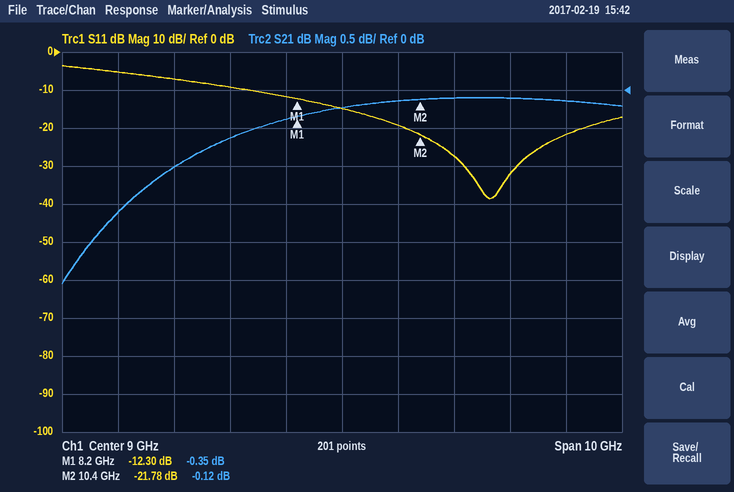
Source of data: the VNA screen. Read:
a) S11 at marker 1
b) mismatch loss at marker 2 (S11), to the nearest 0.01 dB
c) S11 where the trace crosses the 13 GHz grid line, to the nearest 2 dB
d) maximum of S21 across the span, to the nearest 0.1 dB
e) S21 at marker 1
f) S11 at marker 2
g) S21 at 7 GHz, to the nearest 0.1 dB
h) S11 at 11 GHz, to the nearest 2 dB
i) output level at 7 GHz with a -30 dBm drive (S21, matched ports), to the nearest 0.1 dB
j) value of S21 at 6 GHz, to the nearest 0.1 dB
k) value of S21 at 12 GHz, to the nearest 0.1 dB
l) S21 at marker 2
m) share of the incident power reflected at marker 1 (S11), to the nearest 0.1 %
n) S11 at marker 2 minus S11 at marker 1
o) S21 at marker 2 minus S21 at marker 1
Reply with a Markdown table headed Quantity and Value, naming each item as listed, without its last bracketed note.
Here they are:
| Quantity | Value |
|---|---|
| S11 at marker 1 | -12.30 dB |
| mismatch loss at marker 2 (S11), to the nearest 0.01 dB | 0.03 dB |
| S11 where the trace crosses the 13 GHz grid line, to the nearest 2 dB | -22 dB |
| maximum of S21 across the span, to the nearest 0.1 dB | -0.1 dB |
| S21 at marker 1 | -0.35 dB |
| S11 at marker 2 | -21.78 dB |
| S21 at 7 GHz, to the nearest 0.1 dB | -0.6 dB |
| S11 at 11 GHz, to the nearest 2 dB | -28 dB |
| output level at 7 GHz with a -30 dBm drive (S21, matched ports), to the nearest 0.1 dB | -30.6 dBm |
| value of S21 at 6 GHz, to the nearest 0.1 dB | -1.0 dB |
| value of S21 at 12 GHz, to the nearest 0.1 dB | -0.1 dB |
| S21 at marker 2 | -0.12 dB |
| share of the incident power reflected at marker 1 (S11), to the nearest 0.1 % | 5.9 % |
| S11 at marker 2 minus S11 at marker 1 | -9.48 dB |
| S21 at marker 2 minus S21 at marker 1 | 0.23 dB |
